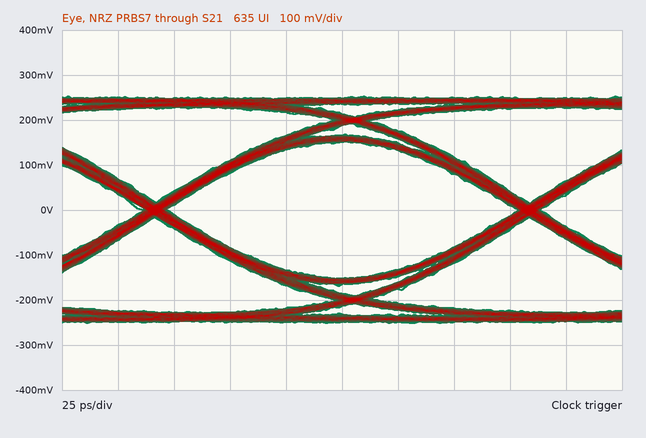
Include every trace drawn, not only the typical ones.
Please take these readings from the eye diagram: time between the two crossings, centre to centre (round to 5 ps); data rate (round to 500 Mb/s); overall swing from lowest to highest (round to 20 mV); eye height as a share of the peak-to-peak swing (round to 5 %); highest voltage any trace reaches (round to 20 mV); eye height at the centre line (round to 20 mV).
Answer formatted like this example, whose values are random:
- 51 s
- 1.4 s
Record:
- 165 ps
- 6.0 Gb/s
- 500 mV
- 60 %
- 260 mV
- 300 mV
